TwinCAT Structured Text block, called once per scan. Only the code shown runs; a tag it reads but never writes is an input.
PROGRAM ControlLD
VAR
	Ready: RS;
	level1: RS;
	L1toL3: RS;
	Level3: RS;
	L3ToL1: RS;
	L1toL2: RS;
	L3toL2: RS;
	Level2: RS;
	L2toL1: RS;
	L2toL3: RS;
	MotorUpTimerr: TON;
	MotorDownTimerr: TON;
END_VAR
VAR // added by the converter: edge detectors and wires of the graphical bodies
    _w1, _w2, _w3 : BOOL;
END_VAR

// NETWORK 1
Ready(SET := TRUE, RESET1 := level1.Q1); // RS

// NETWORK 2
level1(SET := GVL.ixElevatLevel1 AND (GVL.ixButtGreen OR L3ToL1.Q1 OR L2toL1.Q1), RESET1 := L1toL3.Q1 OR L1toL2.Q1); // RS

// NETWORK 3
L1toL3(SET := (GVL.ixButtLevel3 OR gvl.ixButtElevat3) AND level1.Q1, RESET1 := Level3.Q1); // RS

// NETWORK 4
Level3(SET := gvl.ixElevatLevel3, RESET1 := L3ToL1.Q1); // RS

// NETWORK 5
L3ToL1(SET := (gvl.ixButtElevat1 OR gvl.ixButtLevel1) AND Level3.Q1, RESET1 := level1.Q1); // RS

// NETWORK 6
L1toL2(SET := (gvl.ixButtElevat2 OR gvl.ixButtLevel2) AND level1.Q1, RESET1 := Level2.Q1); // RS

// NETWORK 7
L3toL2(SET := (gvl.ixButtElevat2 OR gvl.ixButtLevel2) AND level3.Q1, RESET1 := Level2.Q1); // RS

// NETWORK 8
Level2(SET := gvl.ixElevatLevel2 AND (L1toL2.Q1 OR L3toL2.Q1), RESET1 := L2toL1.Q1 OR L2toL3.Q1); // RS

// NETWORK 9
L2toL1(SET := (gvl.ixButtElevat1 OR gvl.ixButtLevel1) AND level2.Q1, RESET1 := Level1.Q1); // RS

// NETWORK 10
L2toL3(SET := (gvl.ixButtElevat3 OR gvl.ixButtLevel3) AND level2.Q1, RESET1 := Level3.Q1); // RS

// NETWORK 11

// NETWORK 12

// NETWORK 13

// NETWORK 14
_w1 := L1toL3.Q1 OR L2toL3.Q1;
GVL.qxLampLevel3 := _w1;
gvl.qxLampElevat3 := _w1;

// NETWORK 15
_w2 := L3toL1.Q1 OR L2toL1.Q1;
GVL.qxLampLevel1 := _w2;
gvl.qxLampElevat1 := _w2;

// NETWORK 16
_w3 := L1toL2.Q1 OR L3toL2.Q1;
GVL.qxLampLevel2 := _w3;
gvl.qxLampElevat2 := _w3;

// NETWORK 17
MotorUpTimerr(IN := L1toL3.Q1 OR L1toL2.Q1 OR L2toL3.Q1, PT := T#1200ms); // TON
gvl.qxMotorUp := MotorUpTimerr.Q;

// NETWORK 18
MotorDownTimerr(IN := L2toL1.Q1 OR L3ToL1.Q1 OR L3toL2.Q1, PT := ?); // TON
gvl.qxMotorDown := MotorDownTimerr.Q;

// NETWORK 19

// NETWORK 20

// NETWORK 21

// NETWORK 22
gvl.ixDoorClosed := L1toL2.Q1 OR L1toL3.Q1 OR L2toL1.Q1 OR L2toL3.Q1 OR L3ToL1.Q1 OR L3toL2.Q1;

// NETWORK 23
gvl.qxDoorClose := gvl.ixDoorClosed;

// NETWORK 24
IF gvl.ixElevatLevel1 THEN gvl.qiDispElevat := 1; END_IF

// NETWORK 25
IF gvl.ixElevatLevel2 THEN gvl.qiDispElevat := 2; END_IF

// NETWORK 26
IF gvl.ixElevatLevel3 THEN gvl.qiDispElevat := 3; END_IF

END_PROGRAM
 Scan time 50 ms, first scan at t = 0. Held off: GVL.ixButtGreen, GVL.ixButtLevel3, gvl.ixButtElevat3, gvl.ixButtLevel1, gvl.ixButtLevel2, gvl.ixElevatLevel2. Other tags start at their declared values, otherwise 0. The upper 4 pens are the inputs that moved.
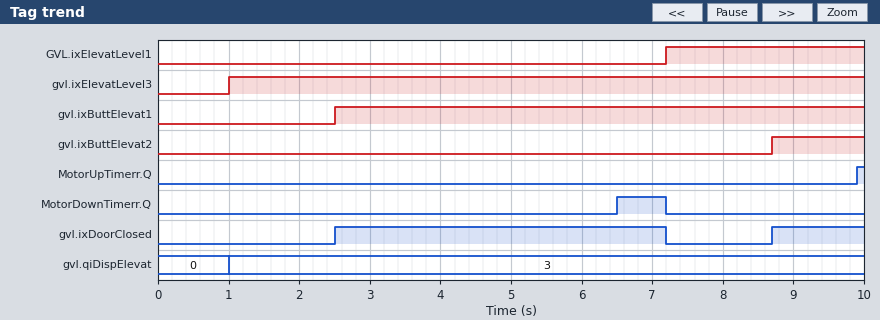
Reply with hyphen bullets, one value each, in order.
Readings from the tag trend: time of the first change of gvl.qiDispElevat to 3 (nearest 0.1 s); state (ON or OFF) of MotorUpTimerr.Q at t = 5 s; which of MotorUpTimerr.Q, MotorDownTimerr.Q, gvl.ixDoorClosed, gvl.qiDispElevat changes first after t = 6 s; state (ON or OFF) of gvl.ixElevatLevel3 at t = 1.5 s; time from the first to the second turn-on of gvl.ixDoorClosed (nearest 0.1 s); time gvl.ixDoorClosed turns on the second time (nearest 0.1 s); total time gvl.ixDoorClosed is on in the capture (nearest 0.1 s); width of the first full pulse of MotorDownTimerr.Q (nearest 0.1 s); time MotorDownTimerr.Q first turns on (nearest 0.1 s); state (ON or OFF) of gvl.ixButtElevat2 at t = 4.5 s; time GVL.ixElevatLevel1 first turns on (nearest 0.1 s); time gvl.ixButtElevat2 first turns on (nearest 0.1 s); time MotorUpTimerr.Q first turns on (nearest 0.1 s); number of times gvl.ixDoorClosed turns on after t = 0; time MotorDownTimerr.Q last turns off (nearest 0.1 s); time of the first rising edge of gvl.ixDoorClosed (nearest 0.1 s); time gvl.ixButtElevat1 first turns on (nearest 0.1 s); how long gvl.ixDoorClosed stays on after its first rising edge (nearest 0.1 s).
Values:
- 1.0 s
- OFF
- MotorDownTimerr.Q
- ON
- 6.2 s
- 8.7 s
- 6.0 s
- 0.7 s
- 6.5 s
- OFF
- 7.2 s
- 8.7 s
- 9.9 s
- 2
- 7.2 s
- 2.5 s
- 2.5 s
- 4.7 s
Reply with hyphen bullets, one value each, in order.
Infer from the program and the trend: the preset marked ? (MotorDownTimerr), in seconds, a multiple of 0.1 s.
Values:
- 4.0 s
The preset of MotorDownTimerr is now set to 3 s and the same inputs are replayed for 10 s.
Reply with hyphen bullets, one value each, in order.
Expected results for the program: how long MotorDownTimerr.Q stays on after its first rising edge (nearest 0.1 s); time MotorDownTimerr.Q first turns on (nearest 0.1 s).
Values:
- 1.7 s
- 5.5 s
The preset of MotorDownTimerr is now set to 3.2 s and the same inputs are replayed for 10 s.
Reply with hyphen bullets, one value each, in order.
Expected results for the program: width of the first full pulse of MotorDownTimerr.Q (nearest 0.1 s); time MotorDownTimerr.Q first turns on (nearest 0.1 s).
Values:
- 1.5 s
- 5.7 s
